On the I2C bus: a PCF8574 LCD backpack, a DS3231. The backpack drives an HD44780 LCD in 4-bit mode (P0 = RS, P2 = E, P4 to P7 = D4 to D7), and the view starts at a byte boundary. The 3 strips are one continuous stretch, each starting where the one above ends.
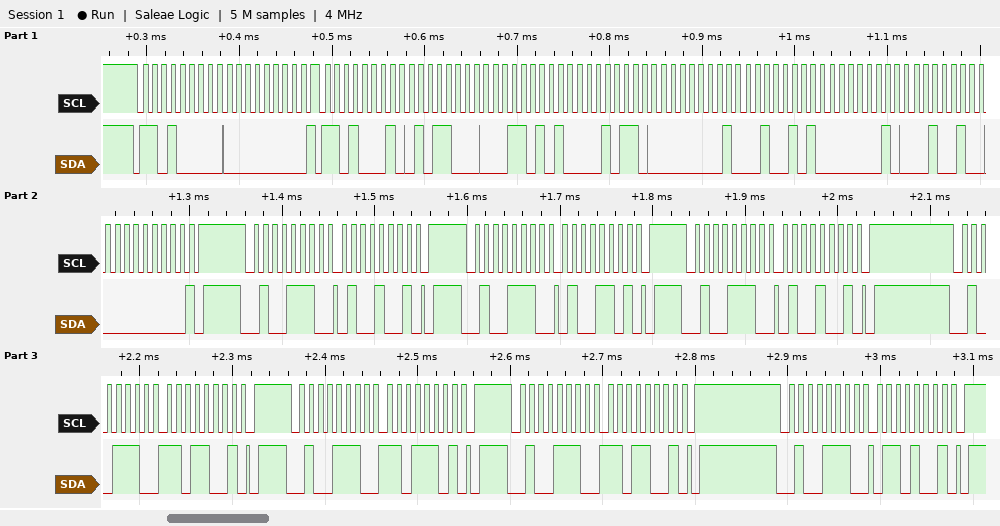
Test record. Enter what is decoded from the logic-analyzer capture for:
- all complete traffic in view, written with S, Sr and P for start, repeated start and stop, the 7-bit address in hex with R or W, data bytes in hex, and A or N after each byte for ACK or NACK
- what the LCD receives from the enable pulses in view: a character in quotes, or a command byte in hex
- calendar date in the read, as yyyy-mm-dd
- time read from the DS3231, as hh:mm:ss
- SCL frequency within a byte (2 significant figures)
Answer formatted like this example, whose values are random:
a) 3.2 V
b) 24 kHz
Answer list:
a) S 68W A 00 A Sr 68R A 58 A 35 A 16 A 01 A 25 A 02 A 24 A 00 N P S 27W A 49 A P S 27W A 4D A P S 27W A 49 A P S 27W A D9 A P S 27W A DD A P S 27W A D9 A P S 27W A 69 A P
b) 'M'
c) 2024-02-25
d) 16:35:58
e) 100 kHz
